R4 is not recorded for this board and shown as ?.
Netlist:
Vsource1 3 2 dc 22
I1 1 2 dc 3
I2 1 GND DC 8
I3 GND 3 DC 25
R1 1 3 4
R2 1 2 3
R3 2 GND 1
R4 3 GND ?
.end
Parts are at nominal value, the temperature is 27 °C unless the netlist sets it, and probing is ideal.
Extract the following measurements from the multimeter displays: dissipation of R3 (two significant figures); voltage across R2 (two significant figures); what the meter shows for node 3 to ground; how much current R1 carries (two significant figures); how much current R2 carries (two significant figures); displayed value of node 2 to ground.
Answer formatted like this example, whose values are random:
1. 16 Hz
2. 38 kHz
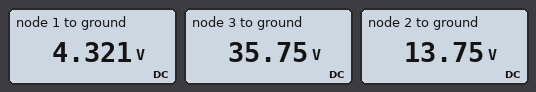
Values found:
1. 190 W
2. 9.4 V
3. 35.75 V
4. 7.9 A
5. 3.1 A
6. 13.75 V
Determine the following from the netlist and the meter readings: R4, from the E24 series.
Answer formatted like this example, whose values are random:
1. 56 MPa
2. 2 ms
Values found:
1. 11 Ω
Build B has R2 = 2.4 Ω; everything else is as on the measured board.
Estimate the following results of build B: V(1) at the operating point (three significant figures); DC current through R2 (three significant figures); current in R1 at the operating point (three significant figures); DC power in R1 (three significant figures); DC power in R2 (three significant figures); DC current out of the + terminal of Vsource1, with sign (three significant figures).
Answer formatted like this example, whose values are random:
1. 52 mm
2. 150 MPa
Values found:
1. 5.50 V
2. 3.44 A
3. 7.56 A
4. 229 W
5. 28.4 W
6. -14.2 A
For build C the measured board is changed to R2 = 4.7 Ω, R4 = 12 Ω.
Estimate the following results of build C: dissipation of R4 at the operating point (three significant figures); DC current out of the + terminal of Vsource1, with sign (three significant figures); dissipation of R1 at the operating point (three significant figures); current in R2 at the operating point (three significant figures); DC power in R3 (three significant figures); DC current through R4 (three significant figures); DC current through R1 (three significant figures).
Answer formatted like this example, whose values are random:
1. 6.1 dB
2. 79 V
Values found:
1. 108 W
2. -13.5 A
3. 287 W
4. 2.53 A
5. 196 W
6. 3.00 A
7. 8.47 A
